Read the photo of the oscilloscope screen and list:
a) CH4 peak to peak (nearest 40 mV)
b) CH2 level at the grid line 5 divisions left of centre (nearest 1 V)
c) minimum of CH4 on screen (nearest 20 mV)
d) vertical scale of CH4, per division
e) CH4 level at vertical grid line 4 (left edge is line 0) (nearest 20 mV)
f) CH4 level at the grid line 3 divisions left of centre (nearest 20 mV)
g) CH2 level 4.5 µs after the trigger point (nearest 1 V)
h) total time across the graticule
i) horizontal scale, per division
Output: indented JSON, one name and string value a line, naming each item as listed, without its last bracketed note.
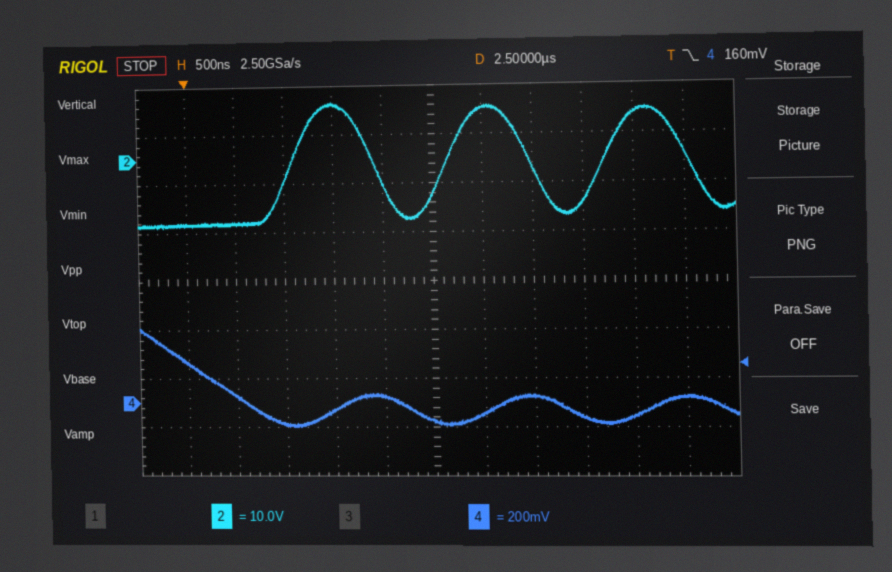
{
  "CH4 peak to peak": "400 mV",
  "CH2 level at the grid line 5 divisions left of centre": "-13 V",
  "minimum of CH4 on screen": "-100 mV",
  "vertical scale of CH4, per division": "200 mV",
  "CH4 level at vertical grid line 4 (left edge is line 0)": "-20 mV",
  "CH4 level at the grid line 3 divisions left of centre": "-80 mV",
  "CH2 level 4.5 µs after the trigger point": "9 V",
  "total time across the graticule": "6 µs",
  "horizontal scale, per division": "500 ns"
}
